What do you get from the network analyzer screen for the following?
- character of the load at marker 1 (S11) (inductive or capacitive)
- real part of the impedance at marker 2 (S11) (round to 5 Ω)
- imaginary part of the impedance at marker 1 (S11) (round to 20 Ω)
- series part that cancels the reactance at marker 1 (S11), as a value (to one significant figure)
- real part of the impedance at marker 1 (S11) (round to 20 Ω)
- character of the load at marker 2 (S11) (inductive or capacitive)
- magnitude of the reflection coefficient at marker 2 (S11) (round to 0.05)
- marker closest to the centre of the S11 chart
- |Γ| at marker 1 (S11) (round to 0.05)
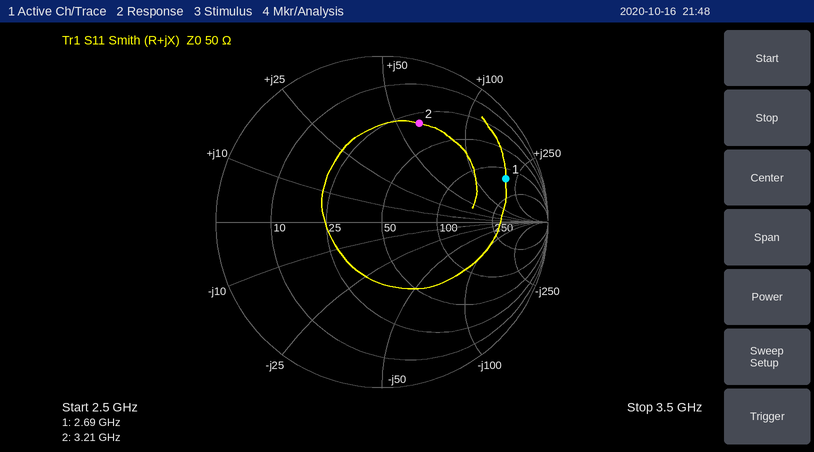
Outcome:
inductive
30 Ω
+200 Ω
300 fF
140 Ω
inductive
0.65
marker 2
0.80
